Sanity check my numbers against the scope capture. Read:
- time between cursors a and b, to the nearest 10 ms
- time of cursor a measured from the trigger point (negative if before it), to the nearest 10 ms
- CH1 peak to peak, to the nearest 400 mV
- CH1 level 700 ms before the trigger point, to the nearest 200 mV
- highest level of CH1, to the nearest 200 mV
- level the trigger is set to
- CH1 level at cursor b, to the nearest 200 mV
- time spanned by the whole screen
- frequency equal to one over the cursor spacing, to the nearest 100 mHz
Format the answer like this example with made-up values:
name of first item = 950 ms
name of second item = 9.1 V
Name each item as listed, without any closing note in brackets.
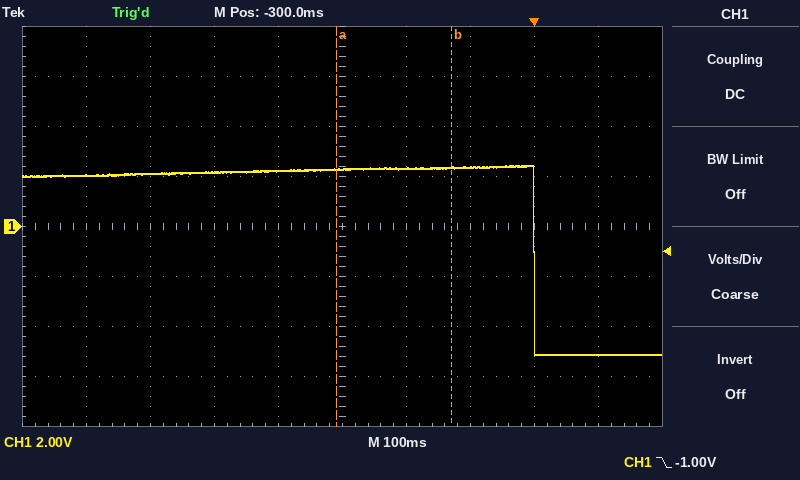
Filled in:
time between cursors a and b, to the nearest 10 ms = 180 ms
time of cursor a measured from the trigger point (negative if before it), to the nearest 10 ms = -310 ms
CH1 peak to peak, to the nearest 400 mV = 7.6 V
CH1 level 700 ms before the trigger point, to the nearest 200 mV = 2.0 V
highest level of CH1, to the nearest 200 mV = 2.4 V
level the trigger is set to = -1.00 V
CH1 level at cursor b, to the nearest 200 mV = 2.4 V
time spanned by the whole screen = 1 s
frequency equal to one over the cursor spacing, to the nearest 100 mHz = 5.6 Hz
